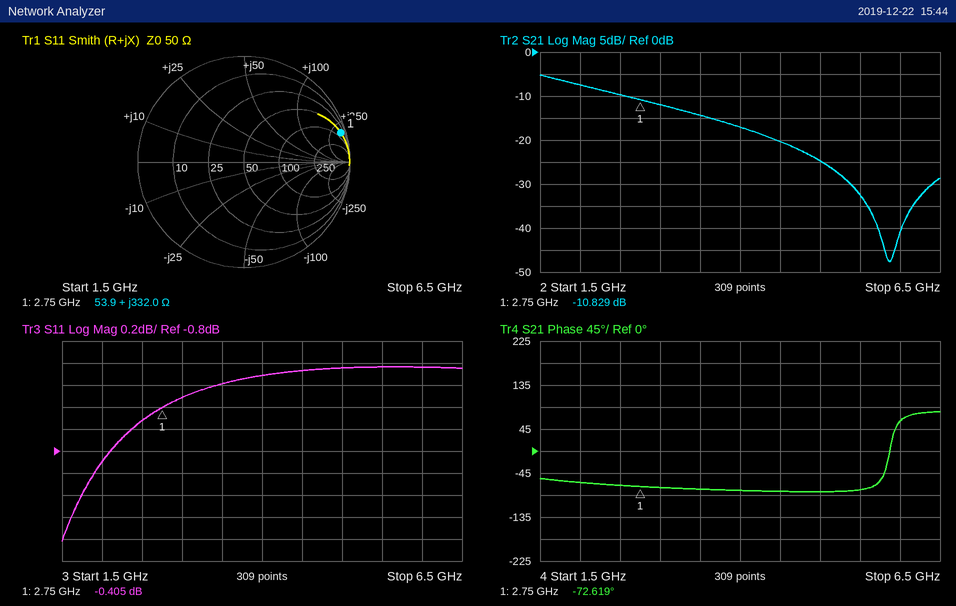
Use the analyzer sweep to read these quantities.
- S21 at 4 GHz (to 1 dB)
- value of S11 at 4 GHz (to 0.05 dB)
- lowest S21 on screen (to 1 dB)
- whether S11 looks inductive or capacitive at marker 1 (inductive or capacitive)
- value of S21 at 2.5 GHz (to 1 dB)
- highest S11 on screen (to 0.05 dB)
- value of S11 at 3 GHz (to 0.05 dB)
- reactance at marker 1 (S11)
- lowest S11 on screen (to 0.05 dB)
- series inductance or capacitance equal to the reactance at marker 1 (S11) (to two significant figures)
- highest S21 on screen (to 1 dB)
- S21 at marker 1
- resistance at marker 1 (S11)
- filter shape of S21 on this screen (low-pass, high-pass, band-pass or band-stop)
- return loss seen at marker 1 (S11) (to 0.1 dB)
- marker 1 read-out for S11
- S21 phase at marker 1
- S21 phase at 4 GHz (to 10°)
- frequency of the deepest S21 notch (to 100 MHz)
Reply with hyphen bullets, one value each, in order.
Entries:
- -17 dB
- -0.10 dB
- -48 dB
- inductive
- -10 dB
- -0.05 dB
- -0.30 dB
- +332.0 Ω
- -1.60 dB
- 19 nH
- -5 dB
- -10.829 dB
- 53.9 Ω
- low-pass
- 0.4 dB
- -0.405 dB
- -72.619°
- -80°
- 5.9 GHz
